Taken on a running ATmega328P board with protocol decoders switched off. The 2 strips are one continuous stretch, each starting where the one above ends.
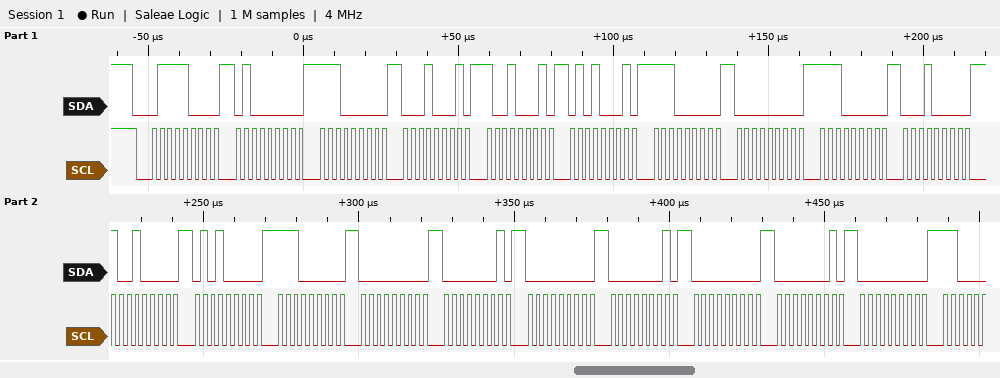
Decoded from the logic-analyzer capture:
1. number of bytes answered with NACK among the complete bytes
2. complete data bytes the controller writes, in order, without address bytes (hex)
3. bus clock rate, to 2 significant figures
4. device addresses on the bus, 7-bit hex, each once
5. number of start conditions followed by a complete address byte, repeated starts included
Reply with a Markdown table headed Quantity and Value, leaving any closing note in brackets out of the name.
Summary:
| Quantity | Value |
|---|---|
| number of bytes answered with NACK among the complete bytes | 0 |
| complete data bytes the controller writes, in order, without address bytes | 40 E0 11 91 51 E0 00 E0 10 90 50 E0 00 01 00 01 00 01 00 |
| bus clock rate, to 2 significant figures | 400 kHz |
| device addresses on the bus, 7-bit hex, each once | 0x3C |
| number of start conditions followed by a complete address byte, repeated starts included | 1 |
